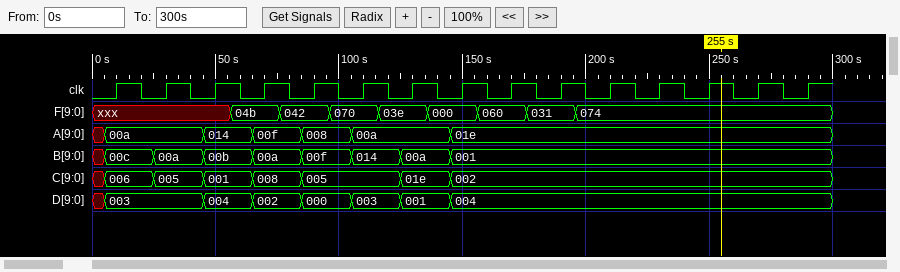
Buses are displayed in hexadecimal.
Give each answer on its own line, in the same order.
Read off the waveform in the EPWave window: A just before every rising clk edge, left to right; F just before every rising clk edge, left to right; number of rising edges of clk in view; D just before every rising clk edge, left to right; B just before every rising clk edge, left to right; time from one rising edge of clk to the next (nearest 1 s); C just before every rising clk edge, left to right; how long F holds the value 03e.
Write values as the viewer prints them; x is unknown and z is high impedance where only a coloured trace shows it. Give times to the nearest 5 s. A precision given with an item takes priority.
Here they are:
00a, 00a, 014, 00f, 008, 00a, 00a, 01e, 01e, 01e, 01e, 01e, 01e, 01e, 01e
xxx, xxx, xxx, 04b, 042, 070, 03e, 000, 060, 031, 074, 074, 074, 074, 074
15
003, 003, 004, 002, 000, 003, 001, 004, 004, 004, 004, 004, 004, 004, 004
00c, 00a, 00b, 00a, 00f, 014, 00a, 001, 001, 001, 001, 001, 001, 001, 001
20 s
006, 005, 001, 008, 005, 005, 01e, 002, 002, 002, 002, 002, 002, 002, 002
20 s
